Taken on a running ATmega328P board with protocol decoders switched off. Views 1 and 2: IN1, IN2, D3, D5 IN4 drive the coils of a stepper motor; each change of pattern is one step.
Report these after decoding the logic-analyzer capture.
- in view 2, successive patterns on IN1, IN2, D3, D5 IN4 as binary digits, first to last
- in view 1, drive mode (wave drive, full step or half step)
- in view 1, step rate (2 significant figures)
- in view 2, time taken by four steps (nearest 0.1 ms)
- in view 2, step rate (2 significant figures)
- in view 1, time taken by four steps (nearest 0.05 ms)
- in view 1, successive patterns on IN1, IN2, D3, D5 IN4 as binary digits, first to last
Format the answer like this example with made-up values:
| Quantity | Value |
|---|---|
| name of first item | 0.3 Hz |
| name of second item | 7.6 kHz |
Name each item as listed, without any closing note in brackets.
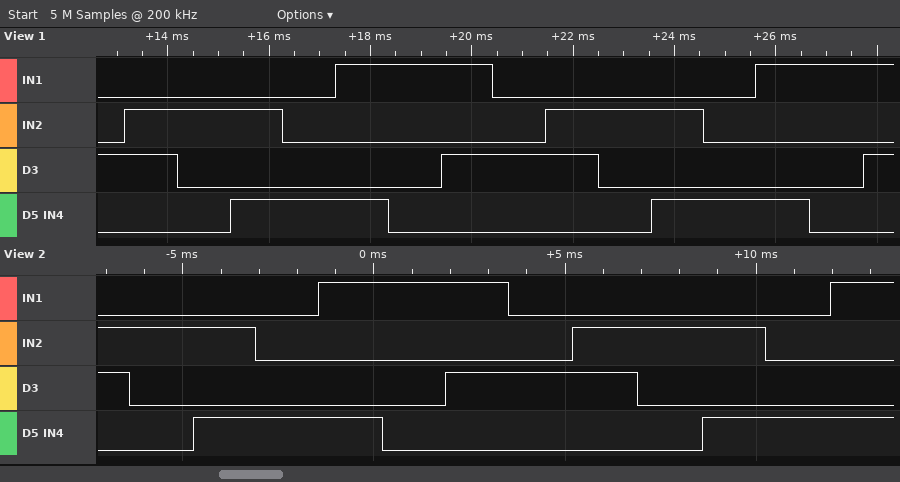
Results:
| Quantity | Value |
|---|---|
| in view 2, successive patterns on IN1, IN2, D3, D5 IN4 as binary digits, first to last | 0110 0100 0101 0001 1001 1000 1010 0010 0110 0100 0101 0001 1001 |
| in view 1, drive mode | half step |
| in view 1, step rate | 960 steps/s |
| in view 2, time taken by four steps | 6.6 ms |
| in view 2, step rate | 600 steps/s |
| in view 1, time taken by four steps | 4.15 ms |
| in view 1, successive patterns on IN1, IN2, D3, D5 IN4 as binary digits, first to last | 0010 0110 0100 0101 0001 1001 1000 1010 0010 0110 0100 0101 0001 1001 1000 1010 |
